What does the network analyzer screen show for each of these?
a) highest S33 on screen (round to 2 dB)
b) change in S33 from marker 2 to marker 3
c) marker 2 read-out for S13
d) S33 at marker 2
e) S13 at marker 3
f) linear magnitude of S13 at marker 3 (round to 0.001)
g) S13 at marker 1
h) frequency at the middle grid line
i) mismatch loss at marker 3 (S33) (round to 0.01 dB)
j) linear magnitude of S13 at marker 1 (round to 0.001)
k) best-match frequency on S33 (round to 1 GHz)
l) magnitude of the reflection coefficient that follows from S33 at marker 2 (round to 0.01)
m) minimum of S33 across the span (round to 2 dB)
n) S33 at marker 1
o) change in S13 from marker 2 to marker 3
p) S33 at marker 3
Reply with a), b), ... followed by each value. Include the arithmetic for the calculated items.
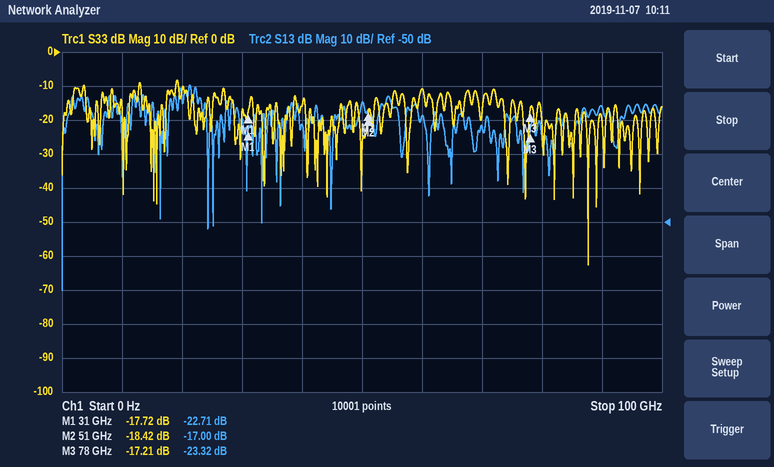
a) -8 dB
b) -17.21 − (-18.42) = 1.21 dB
c) -17.00 dB
d) -18.42 dB
e) -23.32 dB
f) 10^(-23.32/20) ≈ 0.068
g) -22.71 dB
h) 50 GHz
i) −10 log10(1 − 10^(-17.21/10)) ≈ 0.08 dB
j) 10^(-22.71/20) ≈ 0.073
k) 88 GHz
l) 10^(-18.42/20) ≈ 0.12
m) -62 dB
n) -17.72 dB
o) -23.32 − (-17) = -6.32 dB
p) -17.21 dB
